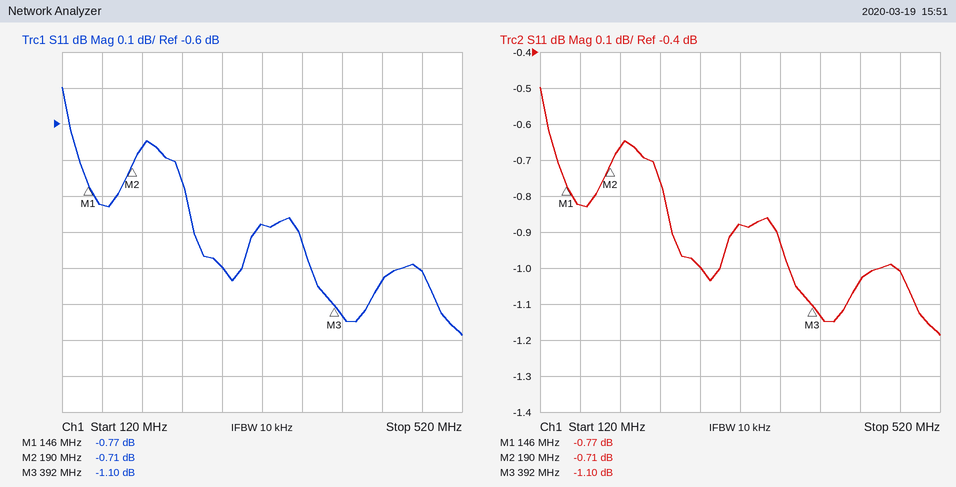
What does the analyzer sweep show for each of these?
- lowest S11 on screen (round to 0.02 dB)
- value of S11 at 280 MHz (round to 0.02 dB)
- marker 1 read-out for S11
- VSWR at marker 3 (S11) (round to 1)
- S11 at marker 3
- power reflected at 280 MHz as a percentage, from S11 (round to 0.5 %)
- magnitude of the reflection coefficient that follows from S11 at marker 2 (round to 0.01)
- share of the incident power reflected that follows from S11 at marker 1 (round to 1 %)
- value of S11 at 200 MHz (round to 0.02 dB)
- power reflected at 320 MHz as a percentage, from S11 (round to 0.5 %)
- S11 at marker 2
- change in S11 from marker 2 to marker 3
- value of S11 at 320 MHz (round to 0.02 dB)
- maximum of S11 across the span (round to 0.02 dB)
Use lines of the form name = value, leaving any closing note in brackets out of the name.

lowest S11 on screen = -1.18 dB
value of S11 at 280 MHz = -1.00 dB
marker 1 read-out for S11 = -0.77 dB
VSWR at marker 3 (S11) = 16
S11 at marker 3 = -1.10 dB
power reflected at 280 MHz as a percentage, from S11 = 79.5 %
magnitude of the reflection coefficient that follows from S11 at marker 2 = 0.92
share of the incident power reflected that follows from S11 at marker 1 = 84 %
value of S11 at 200 MHz = -0.66 dB
power reflected at 320 MHz as a percentage, from S11 = 81.5 %
S11 at marker 2 = -0.71 dB
change in S11 from marker 2 to marker 3 = -0.39 dB
value of S11 at 320 MHz = -0.88 dB
maximum of S11 across the span = -0.50 dB
